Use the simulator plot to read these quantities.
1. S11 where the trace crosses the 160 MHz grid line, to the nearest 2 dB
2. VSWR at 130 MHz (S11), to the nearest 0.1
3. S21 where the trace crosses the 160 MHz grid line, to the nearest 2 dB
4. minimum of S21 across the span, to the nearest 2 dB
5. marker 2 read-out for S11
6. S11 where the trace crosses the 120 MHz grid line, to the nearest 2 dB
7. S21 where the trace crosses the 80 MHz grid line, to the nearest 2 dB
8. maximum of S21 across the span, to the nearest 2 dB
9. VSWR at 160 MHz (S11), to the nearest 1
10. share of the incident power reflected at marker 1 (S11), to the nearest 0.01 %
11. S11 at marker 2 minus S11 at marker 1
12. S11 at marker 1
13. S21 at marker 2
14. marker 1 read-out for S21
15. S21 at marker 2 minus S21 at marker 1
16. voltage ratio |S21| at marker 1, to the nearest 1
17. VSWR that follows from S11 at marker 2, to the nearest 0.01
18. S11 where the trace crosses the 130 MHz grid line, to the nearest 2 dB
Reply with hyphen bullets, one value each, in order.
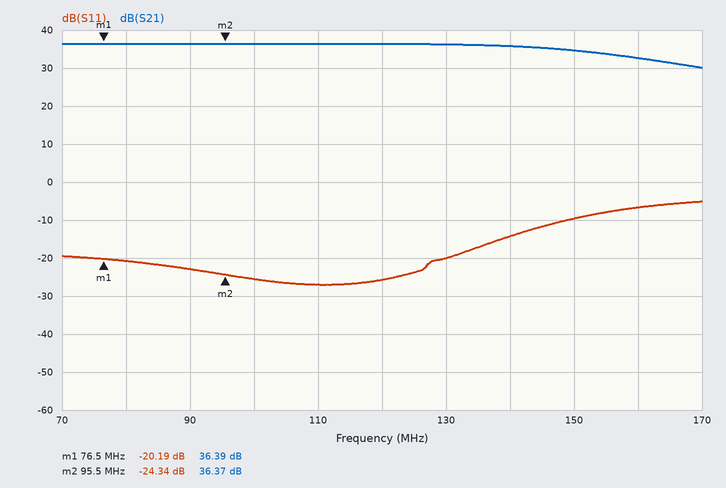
- -6 dB
- 1.2
- 32 dB
- 30 dB
- -24.34 dB
- -26 dB
- 36 dB
- 36 dB
- 3
- 0.96 %
- -4.15 dB
- -20.19 dB
- 36.37 dB
- 36.39 dB
- -0.02 dB
- 66
- 1.13
- -20 dB
